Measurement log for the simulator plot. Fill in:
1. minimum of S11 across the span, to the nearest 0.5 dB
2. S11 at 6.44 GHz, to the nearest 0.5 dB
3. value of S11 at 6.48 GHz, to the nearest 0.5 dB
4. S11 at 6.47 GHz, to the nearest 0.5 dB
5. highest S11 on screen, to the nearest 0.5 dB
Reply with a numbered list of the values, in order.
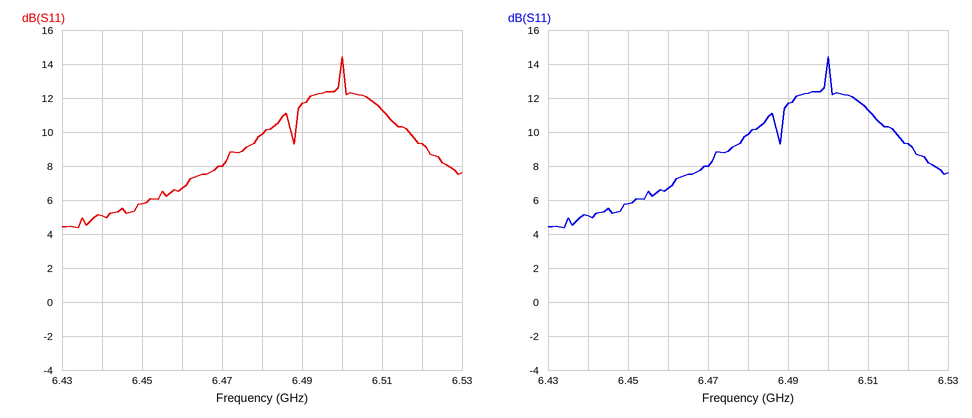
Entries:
1. 4.5 dB
2. 5.0 dB
3. 10.0 dB
4. 8.0 dB
5. 14.5 dB
